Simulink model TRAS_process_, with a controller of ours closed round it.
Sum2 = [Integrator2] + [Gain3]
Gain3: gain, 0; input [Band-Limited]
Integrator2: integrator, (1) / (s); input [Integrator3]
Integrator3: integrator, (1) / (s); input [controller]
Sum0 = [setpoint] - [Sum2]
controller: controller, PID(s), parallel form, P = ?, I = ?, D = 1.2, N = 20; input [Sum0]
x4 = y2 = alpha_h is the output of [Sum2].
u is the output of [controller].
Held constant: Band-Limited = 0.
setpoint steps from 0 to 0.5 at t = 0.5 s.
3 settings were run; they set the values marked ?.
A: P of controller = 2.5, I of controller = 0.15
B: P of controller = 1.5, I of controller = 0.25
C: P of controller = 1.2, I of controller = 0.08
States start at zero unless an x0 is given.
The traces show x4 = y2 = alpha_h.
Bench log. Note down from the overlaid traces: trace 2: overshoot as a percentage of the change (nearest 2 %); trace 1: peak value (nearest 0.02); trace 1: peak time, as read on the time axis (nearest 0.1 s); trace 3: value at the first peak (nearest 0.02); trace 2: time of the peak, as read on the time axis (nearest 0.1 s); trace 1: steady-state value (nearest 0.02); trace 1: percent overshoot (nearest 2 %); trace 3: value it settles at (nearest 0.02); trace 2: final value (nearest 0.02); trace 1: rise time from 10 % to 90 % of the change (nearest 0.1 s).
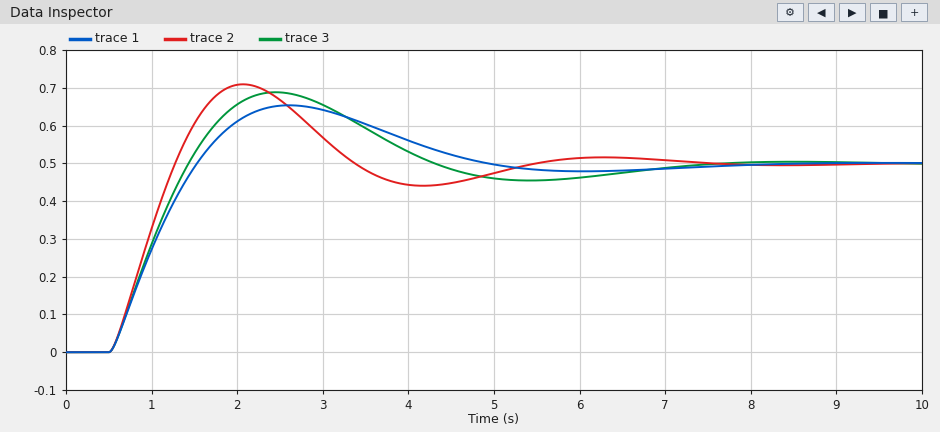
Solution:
42 %
0.66
2.6 s
0.68
2.1 s
0.50
30 %
0.50
0.50
0.8 s
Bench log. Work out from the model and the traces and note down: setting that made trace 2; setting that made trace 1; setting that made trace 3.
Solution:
A
C
B
